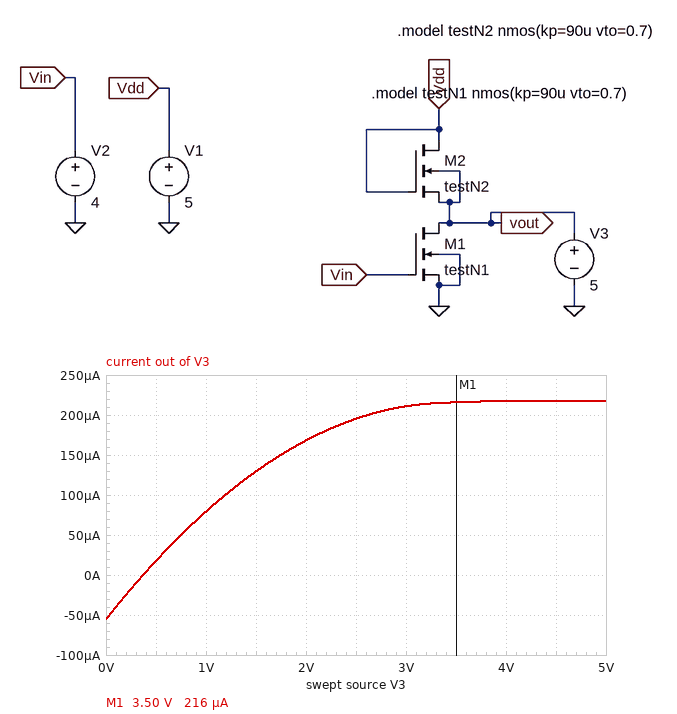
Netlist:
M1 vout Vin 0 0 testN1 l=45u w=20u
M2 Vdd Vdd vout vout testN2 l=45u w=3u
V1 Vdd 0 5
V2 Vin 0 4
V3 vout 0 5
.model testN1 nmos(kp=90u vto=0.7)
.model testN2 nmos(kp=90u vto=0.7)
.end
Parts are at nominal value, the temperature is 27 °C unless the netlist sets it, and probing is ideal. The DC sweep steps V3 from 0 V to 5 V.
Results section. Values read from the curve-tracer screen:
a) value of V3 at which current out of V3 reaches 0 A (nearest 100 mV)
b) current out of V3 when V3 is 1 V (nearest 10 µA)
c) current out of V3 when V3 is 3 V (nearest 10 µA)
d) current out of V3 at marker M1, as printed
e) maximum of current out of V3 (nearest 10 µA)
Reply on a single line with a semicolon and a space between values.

400 mV; 80 µA; 210 µA; 216 µA; 220 µA
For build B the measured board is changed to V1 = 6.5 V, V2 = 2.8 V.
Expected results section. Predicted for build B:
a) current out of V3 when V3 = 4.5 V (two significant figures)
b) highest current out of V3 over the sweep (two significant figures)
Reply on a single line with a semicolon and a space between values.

83 µA; 86 µA
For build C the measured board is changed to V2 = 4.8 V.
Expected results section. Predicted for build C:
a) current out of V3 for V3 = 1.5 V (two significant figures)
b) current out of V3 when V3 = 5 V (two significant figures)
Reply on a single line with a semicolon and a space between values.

180 µA; 340 µA
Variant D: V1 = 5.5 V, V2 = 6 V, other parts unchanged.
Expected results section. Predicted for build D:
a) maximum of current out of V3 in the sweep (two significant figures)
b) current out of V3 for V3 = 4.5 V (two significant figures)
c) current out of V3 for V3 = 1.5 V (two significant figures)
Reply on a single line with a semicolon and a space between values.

560 µA; 550 µA; 240 µA
